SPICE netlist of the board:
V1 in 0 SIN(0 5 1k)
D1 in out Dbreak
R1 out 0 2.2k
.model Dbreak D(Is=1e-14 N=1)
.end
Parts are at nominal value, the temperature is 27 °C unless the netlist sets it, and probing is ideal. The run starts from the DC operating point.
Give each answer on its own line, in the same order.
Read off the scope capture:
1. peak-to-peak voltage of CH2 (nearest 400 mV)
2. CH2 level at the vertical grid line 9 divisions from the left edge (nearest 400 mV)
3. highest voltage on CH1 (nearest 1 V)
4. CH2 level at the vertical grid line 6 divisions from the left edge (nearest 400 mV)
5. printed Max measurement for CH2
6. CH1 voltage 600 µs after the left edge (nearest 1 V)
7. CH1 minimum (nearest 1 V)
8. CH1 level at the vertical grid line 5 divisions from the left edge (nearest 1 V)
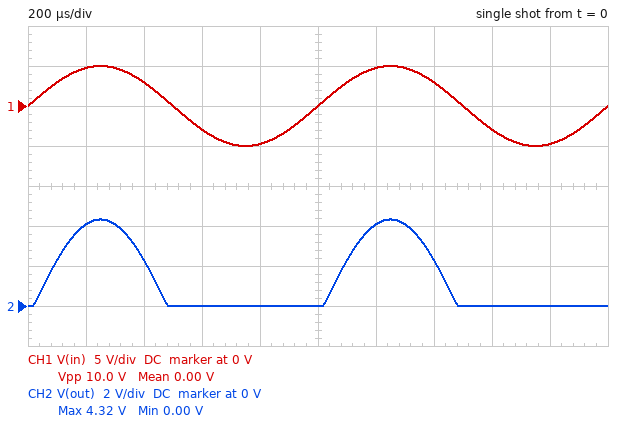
4.4 V
0 V
5 V
4.0 V
4.32 V
-3 V
-5 V
0 V
